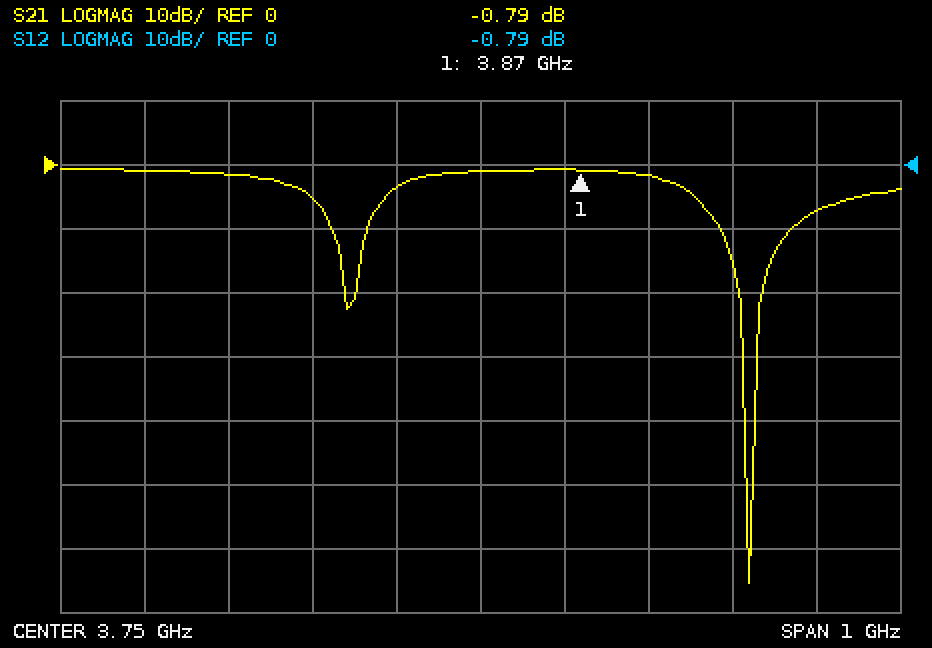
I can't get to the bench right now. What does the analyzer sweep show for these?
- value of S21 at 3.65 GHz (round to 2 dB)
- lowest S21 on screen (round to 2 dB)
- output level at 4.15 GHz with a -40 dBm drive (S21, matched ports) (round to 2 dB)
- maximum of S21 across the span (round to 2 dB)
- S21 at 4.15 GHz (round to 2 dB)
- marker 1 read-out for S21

-4 dB
-66 dB
-48 dBm
0 dB
-8 dB
-0.79 dB
